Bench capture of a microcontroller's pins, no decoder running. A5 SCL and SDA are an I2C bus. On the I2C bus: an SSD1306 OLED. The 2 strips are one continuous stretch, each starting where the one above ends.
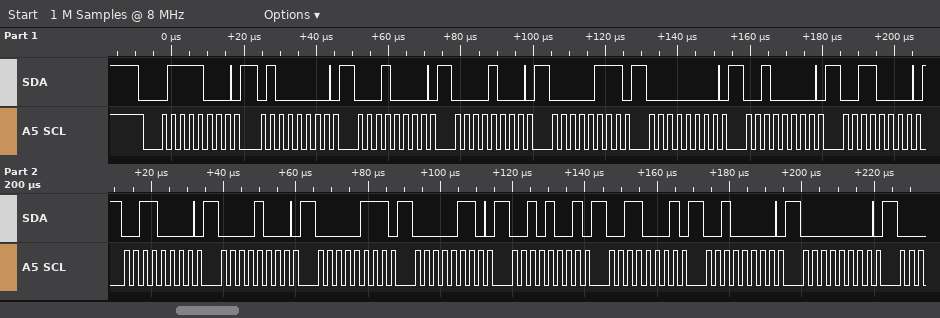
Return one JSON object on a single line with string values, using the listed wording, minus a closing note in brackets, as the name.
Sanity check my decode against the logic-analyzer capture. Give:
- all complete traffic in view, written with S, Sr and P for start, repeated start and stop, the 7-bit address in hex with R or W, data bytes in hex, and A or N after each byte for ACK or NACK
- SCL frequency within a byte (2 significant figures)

{"all complete traffic in view, written with S, Sr and P for start, repeated start and stop, the 7-bit address in hex with R or W, data bytes in hex, and A or N after each byte for ACK or NACK": "S 3CW A 40 A 10 A 08 A 07 A 00 A 20 A 30 A 30 A 08 A 07 A 06 A 29 A 31 A 20 A 00 A", "SCL frequency within a byte": "400 kHz"}
